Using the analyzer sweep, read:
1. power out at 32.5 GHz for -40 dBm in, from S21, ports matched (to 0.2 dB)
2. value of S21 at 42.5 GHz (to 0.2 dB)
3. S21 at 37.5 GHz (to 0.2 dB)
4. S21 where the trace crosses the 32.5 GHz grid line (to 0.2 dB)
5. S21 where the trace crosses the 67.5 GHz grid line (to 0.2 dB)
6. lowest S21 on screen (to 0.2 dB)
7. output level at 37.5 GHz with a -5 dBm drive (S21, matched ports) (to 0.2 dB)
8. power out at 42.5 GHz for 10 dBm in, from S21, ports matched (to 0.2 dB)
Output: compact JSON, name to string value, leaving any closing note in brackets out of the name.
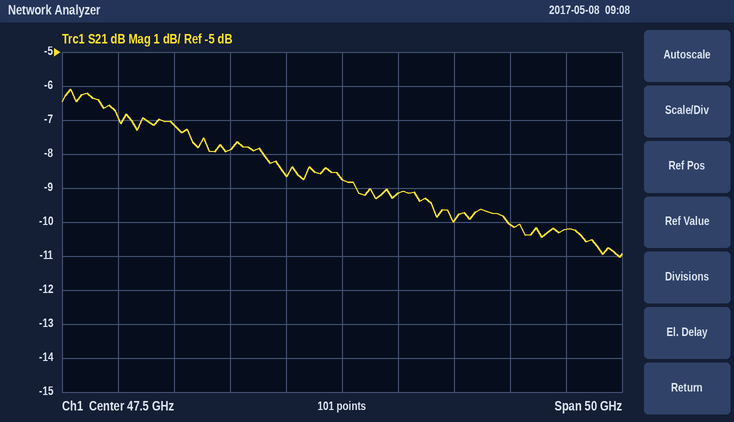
{"power out at 32.5 GHz for -40 dBm in, from S21, ports matched": "-47.2 dBm", "value of S21 at 42.5 GHz": "-8.6 dB", "S21 at 37.5 GHz": "-7.8 dB", "S21 where the trace crosses the 32.5 GHz grid line": "-7.2 dB", "S21 where the trace crosses the 67.5 GHz grid line": "-10.2 dB", "lowest S21 on screen": "-11.0 dB", "output level at 37.5 GHz with a -5 dBm drive (S21, matched ports)": "-12.8 dBm", "power out at 42.5 GHz for 10 dBm in, from S21, ports matched": "1.4 dBm"}
